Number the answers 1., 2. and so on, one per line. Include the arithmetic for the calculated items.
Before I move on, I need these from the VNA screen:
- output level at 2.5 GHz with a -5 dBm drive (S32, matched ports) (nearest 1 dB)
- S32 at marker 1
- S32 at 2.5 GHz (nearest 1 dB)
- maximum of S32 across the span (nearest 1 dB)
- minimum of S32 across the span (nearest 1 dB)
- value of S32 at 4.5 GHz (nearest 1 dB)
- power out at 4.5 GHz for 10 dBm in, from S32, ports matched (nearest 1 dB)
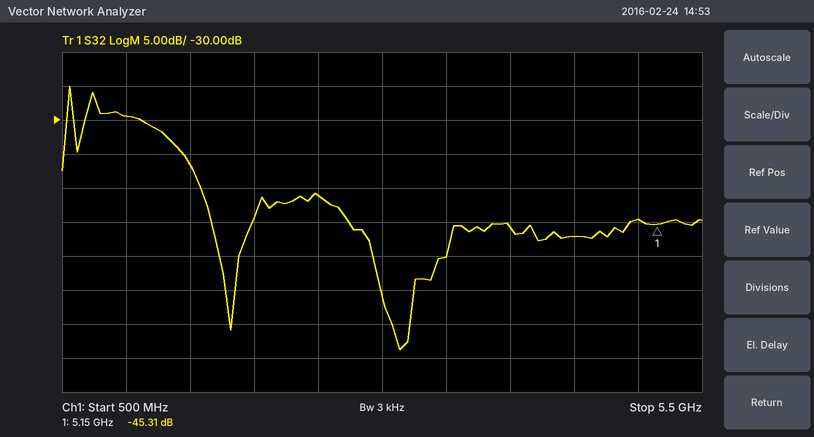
1. -5 dBm + (-41 dB) = -46 dBm
2. -45.31 dB
3. -41 dB
4. -25 dB
5. -64 dB
6. -47 dB
7. 10 dBm + (-47 dB) = -37 dBm
